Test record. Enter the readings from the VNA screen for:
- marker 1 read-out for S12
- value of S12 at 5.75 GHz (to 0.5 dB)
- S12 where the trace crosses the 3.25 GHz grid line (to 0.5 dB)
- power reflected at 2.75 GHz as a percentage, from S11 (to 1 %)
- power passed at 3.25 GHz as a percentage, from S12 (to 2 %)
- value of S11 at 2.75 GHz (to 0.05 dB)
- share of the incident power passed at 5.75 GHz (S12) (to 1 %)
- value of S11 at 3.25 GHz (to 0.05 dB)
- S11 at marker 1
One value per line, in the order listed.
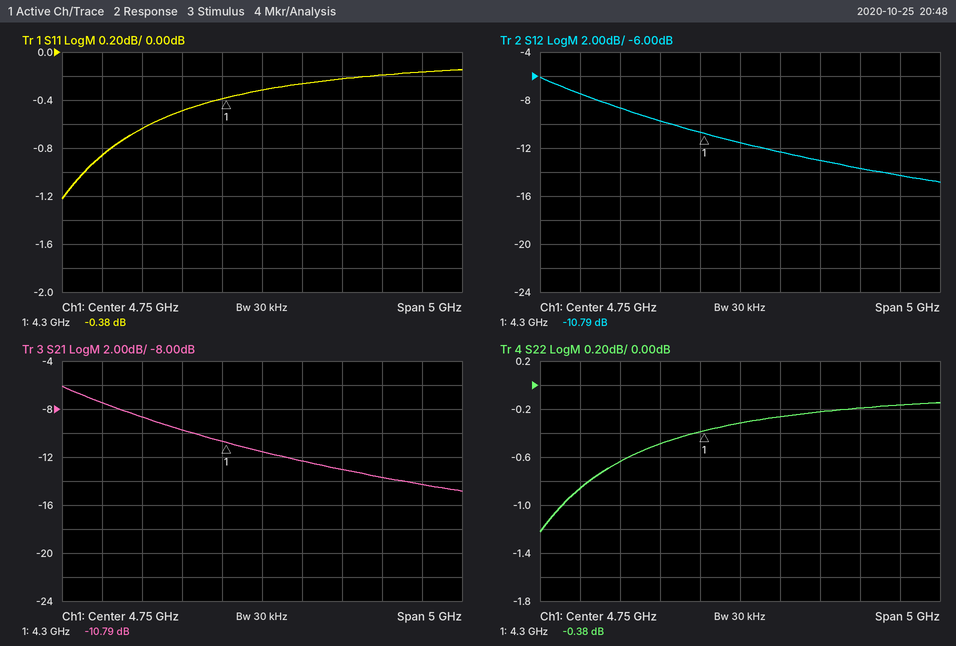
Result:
-10.79 dB
-13.0 dB
-8.5 dB
82 %
14 %
-0.85 dB
5 %
-0.65 dB
-0.38 dB
